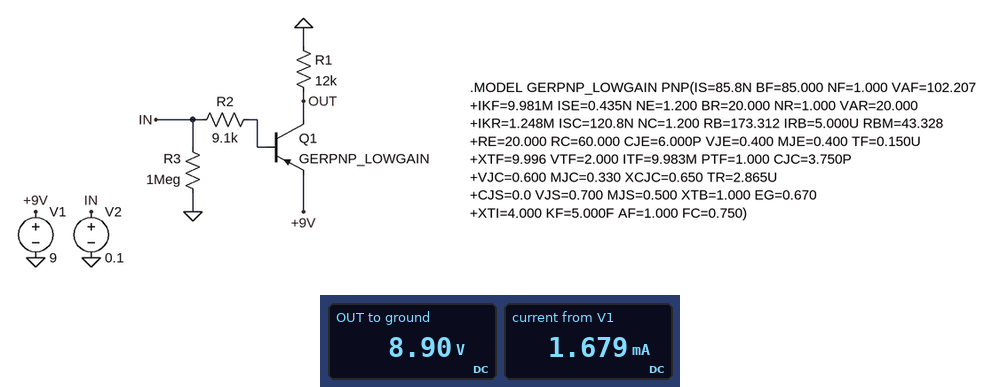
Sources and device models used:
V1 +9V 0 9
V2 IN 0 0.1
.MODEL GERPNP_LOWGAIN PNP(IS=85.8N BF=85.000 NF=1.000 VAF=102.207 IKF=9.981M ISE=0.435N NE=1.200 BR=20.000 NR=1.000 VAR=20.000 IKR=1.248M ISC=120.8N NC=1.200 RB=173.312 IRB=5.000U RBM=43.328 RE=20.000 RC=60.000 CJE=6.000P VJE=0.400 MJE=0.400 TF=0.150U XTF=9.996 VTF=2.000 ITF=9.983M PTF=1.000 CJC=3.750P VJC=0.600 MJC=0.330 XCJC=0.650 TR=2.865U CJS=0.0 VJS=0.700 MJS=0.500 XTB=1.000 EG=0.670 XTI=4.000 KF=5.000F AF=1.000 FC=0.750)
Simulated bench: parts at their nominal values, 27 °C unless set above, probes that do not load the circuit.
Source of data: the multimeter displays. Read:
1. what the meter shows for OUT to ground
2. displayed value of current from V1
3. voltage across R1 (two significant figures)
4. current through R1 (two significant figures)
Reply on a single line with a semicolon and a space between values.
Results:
8.90 V; 1.679 mA; 8.9 V; 740 µA
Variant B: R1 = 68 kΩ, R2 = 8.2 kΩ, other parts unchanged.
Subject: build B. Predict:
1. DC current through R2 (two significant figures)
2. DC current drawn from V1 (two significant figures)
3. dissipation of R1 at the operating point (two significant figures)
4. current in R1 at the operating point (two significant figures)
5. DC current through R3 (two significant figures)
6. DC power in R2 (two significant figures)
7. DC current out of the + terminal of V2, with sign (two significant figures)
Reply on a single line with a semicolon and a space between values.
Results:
1.0 mA; 1.2 mA; 1.2 mW; 130 µA; 100 nA; 8.9 mW; -1.0 mA
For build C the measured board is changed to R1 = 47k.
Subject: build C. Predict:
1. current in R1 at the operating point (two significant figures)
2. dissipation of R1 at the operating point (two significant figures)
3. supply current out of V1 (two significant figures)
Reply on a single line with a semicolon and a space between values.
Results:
190 µA; 1.7 mW; 1.1 mA
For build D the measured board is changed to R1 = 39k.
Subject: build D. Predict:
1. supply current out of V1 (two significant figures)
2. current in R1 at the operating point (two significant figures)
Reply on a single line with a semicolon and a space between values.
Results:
1.2 mA; 230 µA
